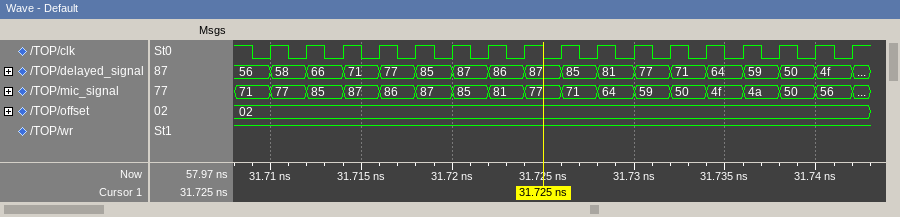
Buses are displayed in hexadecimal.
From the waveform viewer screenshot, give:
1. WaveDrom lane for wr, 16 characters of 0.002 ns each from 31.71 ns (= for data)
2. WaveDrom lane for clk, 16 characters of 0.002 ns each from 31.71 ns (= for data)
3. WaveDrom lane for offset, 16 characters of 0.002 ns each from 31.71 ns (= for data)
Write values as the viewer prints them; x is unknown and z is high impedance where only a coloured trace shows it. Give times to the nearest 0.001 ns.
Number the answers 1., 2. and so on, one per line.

1. {name: 'wr', wave: '1...............'}
2. {name: 'clk', wave: 'p...............'}
3. {name: 'offset', wave: '=...............', data: '02'}
